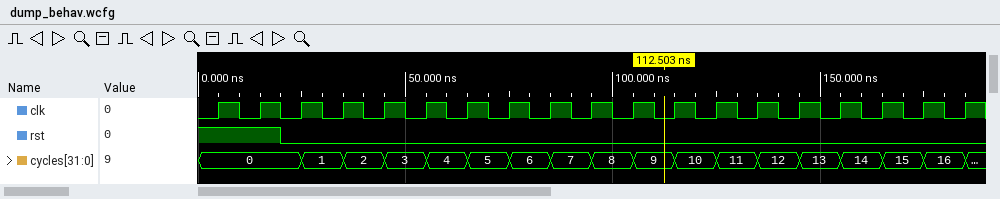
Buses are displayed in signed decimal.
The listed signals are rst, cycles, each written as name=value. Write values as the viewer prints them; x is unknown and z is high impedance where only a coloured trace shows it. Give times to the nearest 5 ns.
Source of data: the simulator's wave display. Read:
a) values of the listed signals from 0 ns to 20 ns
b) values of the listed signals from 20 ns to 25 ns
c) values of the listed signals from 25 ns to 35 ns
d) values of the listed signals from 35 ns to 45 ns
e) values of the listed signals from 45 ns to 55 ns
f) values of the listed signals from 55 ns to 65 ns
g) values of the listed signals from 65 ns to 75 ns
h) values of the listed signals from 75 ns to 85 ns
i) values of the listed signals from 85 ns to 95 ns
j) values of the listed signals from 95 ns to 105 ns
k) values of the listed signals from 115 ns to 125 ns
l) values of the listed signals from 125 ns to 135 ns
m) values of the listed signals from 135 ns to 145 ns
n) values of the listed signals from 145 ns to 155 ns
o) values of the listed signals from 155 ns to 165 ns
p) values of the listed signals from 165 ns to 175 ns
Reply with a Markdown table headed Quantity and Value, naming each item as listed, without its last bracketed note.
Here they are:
| Quantity | Value |
|---|---|
| values of the listed signals from 0 ns to 20 ns | rst=1, cycles=0 |
| values of the listed signals from 20 ns to 25 ns | rst=0, cycles=0 |
| values of the listed signals from 25 ns to 35 ns | rst=0, cycles=1 |
| values of the listed signals from 35 ns to 45 ns | rst=0, cycles=2 |
| values of the listed signals from 45 ns to 55 ns | rst=0, cycles=3 |
| values of the listed signals from 55 ns to 65 ns | rst=0, cycles=4 |
| values of the listed signals from 65 ns to 75 ns | rst=0, cycles=5 |
| values of the listed signals from 75 ns to 85 ns | rst=0, cycles=6 |
| values of the listed signals from 85 ns to 95 ns | rst=0, cycles=7 |
| values of the listed signals from 95 ns to 105 ns | rst=0, cycles=8 |
| values of the listed signals from 115 ns to 125 ns | rst=0, cycles=10 |
| values of the listed signals from 125 ns to 135 ns | rst=0, cycles=11 |
| values of the listed signals from 135 ns to 145 ns | rst=0, cycles=12 |
| values of the listed signals from 145 ns to 155 ns | rst=0, cycles=13 |
| values of the listed signals from 155 ns to 165 ns | rst=0, cycles=14 |
| values of the listed signals from 165 ns to 175 ns | rst=0, cycles=15 |
